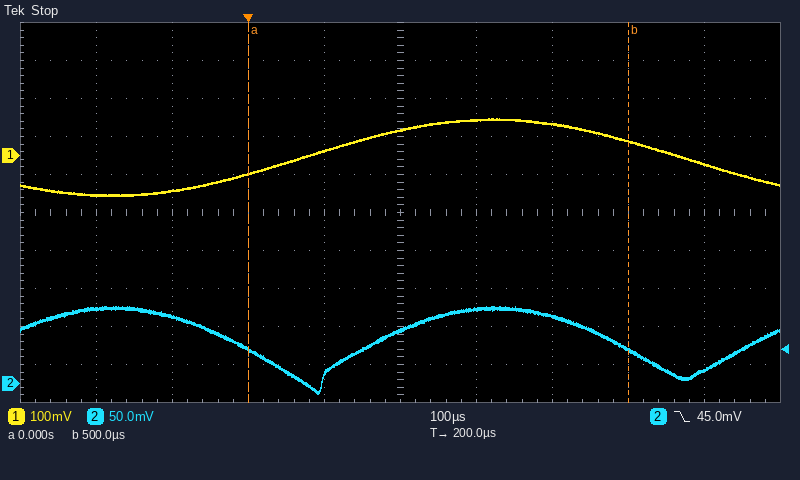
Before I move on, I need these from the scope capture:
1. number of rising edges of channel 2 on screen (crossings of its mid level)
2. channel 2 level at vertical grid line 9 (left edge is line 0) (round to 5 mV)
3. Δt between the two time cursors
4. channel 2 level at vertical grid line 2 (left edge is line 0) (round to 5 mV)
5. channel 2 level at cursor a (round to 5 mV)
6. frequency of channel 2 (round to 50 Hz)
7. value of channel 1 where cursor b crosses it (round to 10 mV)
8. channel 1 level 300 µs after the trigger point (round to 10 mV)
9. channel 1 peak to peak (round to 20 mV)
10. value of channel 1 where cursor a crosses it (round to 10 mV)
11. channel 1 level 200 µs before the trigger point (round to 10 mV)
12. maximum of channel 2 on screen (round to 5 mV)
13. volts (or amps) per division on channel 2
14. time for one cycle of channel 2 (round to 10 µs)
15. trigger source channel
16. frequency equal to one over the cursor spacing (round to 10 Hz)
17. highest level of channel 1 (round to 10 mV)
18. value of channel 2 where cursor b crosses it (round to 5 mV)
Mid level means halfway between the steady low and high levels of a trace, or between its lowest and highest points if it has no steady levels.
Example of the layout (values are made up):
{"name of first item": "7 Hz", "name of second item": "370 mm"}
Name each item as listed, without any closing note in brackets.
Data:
{"number of rising edges of channel 2 on screen": "2", "channel 2 level at vertical grid line 9 (left edge is line 0)": "20 mV", "Δt between the two time cursors": "500 µs", "channel 2 level at vertical grid line 2 (left edge is line 0)": "90 mV", "channel 2 level at cursor a": "45 mV", "frequency of channel 2": "2.00 kHz", "value of channel 1 where cursor b crosses it": "40 mV", "channel 1 level 300 µs after the trigger point": "90 mV", "channel 1 peak to peak": "200 mV", "value of channel 1 where cursor a crosses it": "-50 mV", "channel 1 level 200 µs before the trigger point": "-100 mV", "maximum of channel 2 on screen": "100 mV", "volts (or amps) per division on channel 2": "50 mV", "time for one cycle of channel 2": "500 µs", "trigger source channel": "channel 2", "frequency equal to one over the cursor spacing": "2.00 kHz", "highest level of channel 1": "100 mV", "value of channel 2 where cursor b crosses it": "45 mV"}
